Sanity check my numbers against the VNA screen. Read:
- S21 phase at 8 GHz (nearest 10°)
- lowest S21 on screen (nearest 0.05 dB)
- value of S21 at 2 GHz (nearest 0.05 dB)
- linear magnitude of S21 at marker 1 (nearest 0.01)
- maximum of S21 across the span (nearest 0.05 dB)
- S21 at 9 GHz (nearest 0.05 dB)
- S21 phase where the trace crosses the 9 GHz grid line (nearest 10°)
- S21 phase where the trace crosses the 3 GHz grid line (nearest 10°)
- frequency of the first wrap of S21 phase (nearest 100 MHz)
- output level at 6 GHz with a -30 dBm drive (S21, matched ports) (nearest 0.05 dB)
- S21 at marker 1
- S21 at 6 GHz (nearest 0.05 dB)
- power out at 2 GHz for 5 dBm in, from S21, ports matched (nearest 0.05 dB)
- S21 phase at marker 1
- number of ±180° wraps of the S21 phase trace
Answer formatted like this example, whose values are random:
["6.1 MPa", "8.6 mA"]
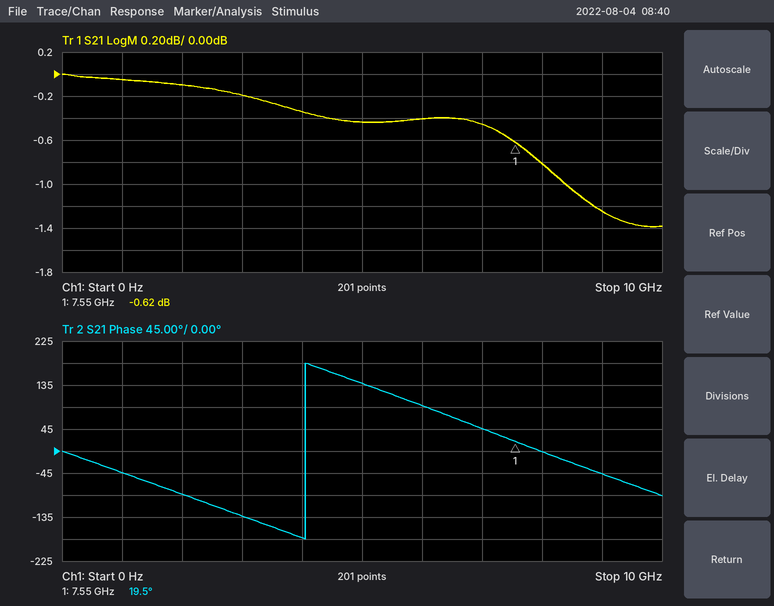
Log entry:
["0°", "-1.40 dB", "-0.10 dB", "0.93", "0.00 dB", "-1.25 dB", "-50°", "-130°", "4.1 GHz", "-30.40 dBm", "-0.62 dB", "-0.40 dB", "4.90 dBm", "19.5°", "1"]
